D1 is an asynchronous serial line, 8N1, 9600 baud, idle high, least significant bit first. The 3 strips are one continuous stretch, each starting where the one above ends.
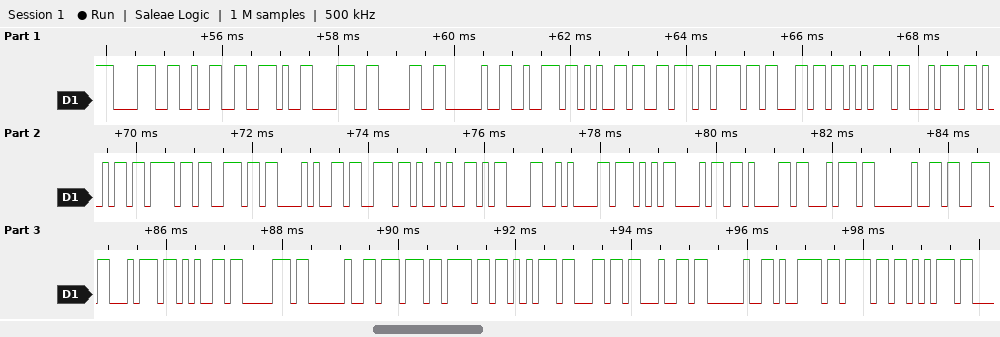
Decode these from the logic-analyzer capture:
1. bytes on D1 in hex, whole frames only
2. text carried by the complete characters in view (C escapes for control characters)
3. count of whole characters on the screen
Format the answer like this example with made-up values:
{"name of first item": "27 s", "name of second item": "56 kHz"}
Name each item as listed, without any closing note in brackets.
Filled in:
{"bytes on D1 in hex, whole frames only": "38 32 2E 38 30 20 72 65 76 6F 6C 75 74 69 6F 6E 28 73 29 0D 0A 57 68 61 74 20 73 74 65 70 20 77 6F 75 6C 64 20 79 6F 75", "text carried by the complete characters in view": "\"82.80 revolution(s)\\r\\nWhat step would you\"", "count of whole characters on the screen": "40"}
